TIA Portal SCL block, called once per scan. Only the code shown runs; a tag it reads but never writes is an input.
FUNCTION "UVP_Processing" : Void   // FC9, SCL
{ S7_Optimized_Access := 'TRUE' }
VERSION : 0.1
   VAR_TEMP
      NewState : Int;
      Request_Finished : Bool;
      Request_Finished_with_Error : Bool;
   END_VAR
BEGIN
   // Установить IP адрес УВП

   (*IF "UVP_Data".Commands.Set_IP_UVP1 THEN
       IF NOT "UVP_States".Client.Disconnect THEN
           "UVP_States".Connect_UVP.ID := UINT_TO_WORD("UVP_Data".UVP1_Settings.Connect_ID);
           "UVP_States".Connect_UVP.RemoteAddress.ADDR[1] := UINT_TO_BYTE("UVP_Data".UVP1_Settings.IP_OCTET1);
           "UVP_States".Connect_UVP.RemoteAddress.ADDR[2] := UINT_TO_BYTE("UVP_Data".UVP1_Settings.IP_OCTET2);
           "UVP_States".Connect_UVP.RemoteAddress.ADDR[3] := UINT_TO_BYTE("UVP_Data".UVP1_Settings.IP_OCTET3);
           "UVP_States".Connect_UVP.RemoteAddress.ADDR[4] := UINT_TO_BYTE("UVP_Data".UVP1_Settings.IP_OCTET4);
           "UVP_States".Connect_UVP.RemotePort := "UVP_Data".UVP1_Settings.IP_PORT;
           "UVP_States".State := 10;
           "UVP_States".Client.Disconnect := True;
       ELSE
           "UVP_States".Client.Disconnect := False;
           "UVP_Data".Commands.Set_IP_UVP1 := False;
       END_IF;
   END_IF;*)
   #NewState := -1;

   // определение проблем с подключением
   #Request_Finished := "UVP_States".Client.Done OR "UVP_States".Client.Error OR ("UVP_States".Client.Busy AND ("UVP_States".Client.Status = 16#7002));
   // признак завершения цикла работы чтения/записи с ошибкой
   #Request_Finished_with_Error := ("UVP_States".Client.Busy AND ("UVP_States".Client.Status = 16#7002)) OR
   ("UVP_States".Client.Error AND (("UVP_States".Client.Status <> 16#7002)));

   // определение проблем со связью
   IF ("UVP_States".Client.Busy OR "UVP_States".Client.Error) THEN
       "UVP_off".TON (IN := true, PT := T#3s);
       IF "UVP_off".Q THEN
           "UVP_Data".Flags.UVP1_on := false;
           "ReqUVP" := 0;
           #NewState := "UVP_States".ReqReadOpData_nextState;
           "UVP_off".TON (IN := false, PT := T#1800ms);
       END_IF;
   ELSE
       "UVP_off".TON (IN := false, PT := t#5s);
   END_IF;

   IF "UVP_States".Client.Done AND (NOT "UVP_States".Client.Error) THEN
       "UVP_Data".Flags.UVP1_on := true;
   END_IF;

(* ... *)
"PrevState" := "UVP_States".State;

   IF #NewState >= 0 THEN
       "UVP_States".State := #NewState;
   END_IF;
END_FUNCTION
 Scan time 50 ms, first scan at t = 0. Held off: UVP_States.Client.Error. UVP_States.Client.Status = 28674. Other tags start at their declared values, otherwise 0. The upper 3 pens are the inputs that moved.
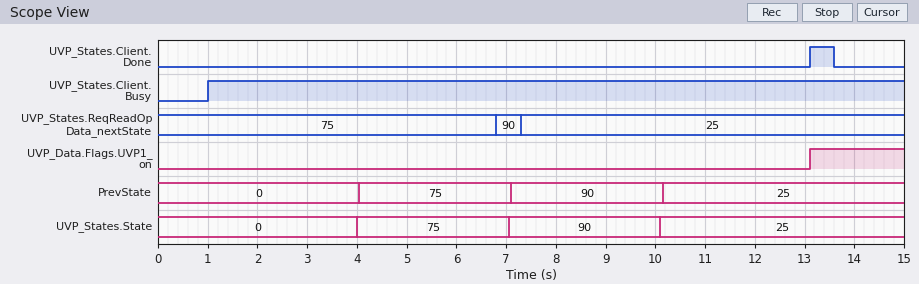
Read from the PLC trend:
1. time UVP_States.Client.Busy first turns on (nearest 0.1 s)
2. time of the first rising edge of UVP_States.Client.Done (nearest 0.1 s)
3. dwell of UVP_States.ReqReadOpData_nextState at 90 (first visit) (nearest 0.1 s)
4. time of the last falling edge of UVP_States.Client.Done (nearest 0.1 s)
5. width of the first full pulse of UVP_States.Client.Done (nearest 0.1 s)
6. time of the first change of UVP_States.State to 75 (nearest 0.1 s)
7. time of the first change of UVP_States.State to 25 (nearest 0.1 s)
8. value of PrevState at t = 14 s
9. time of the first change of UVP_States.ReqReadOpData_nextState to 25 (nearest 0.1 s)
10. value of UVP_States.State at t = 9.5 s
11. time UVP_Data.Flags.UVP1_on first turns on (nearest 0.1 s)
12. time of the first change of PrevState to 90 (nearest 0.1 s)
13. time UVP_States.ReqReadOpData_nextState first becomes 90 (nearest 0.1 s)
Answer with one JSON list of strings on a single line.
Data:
["1.0 s", "13.1 s", "0.5 s", "13.6 s", "0.5 s", "4.0 s", "10.1 s", "25", "7.3 s", "90", "13.1 s", "7.1 s", "6.8 s"]
